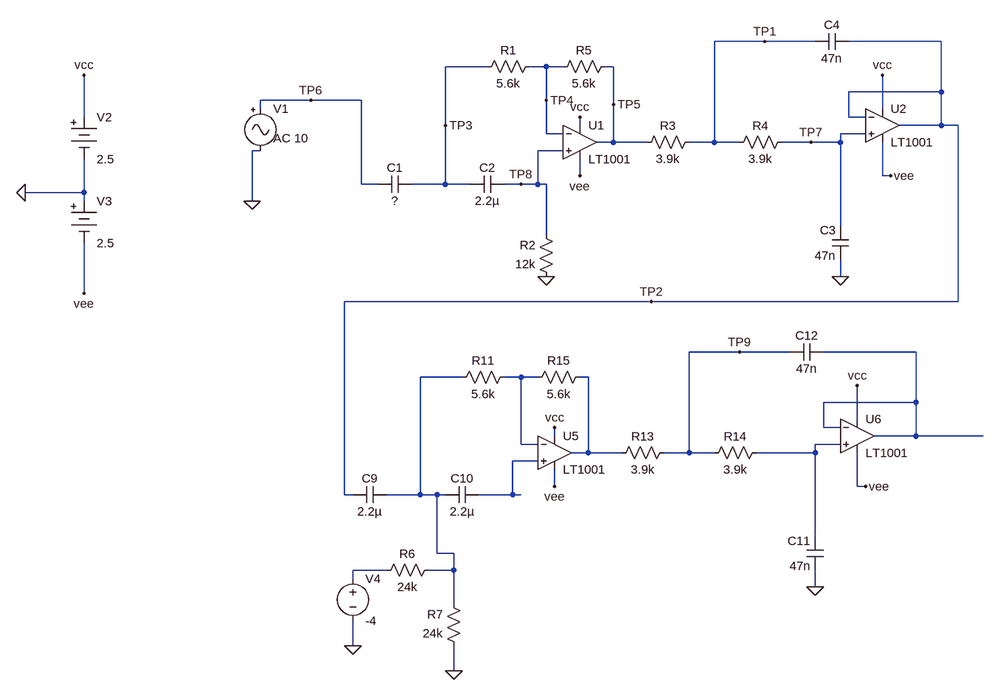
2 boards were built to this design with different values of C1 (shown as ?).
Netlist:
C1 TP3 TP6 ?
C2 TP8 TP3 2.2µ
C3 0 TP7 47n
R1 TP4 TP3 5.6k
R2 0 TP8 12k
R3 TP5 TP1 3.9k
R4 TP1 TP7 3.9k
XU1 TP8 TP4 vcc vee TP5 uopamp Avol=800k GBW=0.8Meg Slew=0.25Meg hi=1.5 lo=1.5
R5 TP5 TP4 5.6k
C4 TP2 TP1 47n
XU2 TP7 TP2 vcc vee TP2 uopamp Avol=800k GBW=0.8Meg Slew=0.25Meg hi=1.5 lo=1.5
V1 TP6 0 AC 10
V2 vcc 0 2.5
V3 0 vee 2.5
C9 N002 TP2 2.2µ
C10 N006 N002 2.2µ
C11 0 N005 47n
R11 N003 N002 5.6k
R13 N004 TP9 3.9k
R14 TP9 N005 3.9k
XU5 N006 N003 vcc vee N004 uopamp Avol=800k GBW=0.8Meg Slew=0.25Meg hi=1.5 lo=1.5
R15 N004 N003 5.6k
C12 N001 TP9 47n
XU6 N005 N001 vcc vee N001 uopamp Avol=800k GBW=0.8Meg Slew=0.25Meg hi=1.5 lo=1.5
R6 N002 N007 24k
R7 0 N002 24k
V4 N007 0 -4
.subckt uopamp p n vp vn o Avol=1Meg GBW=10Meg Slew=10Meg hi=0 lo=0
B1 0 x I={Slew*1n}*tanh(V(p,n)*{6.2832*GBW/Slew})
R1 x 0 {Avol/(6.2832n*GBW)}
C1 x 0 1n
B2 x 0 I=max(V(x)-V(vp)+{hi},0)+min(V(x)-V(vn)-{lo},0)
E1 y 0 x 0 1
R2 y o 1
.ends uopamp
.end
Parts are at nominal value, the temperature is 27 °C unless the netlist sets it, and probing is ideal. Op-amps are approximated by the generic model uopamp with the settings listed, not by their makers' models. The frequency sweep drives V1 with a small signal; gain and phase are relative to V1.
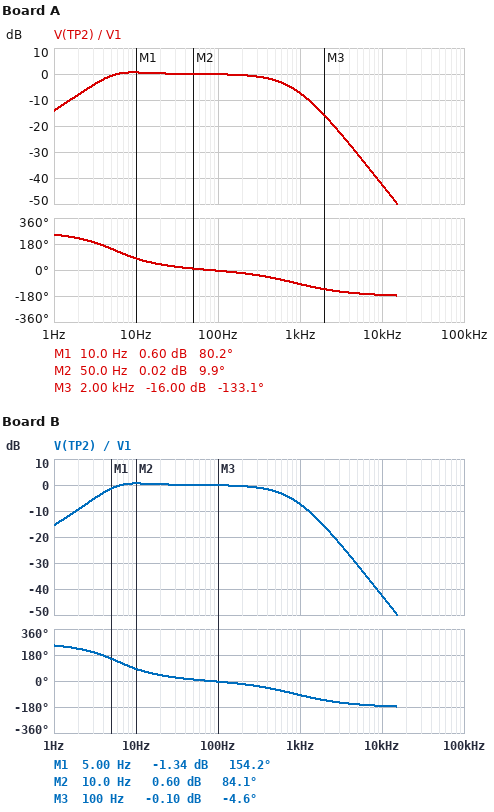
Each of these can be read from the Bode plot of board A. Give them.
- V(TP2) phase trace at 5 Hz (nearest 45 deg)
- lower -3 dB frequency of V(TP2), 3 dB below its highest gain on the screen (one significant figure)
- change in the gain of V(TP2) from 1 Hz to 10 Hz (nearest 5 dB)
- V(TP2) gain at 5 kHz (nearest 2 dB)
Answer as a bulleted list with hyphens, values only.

- 135 deg
- 4 Hz
- 15 dB
- -30 dB
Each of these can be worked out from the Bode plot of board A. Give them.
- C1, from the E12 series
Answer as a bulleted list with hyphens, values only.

- 5.6 µF
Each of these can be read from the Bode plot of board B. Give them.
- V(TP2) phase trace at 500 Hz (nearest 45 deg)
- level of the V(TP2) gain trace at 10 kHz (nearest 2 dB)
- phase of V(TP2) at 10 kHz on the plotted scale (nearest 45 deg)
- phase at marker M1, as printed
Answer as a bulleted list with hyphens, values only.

- -45 deg
- -42 dB
- -180 deg
- 154.2 deg
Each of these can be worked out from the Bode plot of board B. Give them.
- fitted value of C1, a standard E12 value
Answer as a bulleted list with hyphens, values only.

- 4.7 µF
